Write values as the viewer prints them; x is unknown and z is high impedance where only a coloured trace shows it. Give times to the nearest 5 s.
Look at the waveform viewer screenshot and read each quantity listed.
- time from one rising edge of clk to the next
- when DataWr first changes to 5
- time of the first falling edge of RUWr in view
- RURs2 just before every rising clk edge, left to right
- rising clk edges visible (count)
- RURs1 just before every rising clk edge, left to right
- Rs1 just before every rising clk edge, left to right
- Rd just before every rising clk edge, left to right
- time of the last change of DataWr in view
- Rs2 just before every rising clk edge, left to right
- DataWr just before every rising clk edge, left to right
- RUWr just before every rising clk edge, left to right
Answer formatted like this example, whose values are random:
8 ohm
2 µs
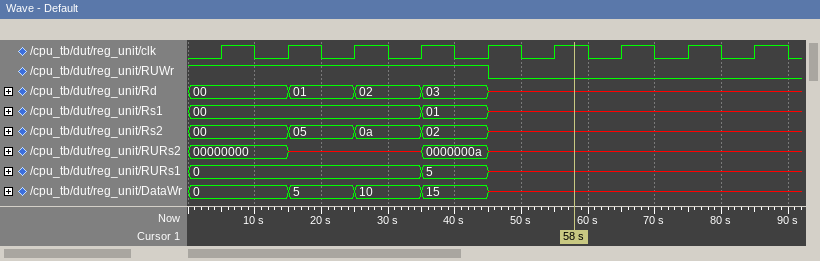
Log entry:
10 s
15 s
45 s
00000000, 00000000, x, x, 0000000a, x, x, x, x
9
0, 0, 0, 0, 5, x, x, x, x
00, 00, 00, 00, 01, x, x, x, x
00, 00, 01, 02, 03, x, x, x, x
45 s
00, 00, 05, 0a, 02, x, x, x, x
0, 0, 5, 10, 15, x, x, x, x
1 1 1 1 1 0 0 0 0
